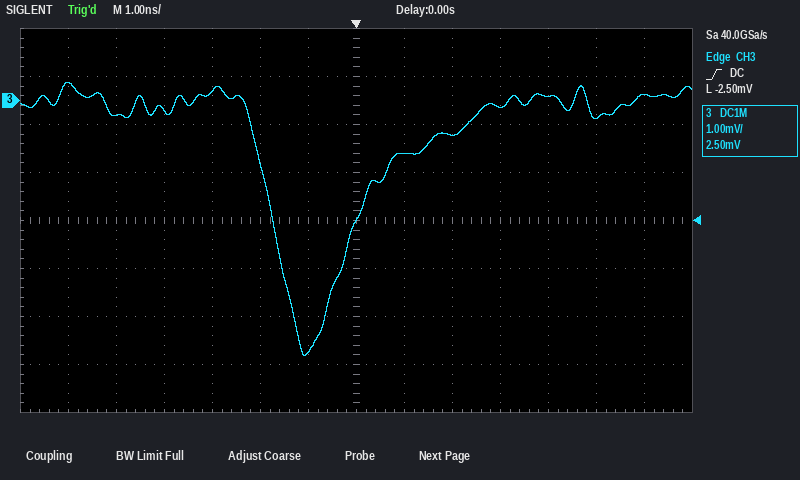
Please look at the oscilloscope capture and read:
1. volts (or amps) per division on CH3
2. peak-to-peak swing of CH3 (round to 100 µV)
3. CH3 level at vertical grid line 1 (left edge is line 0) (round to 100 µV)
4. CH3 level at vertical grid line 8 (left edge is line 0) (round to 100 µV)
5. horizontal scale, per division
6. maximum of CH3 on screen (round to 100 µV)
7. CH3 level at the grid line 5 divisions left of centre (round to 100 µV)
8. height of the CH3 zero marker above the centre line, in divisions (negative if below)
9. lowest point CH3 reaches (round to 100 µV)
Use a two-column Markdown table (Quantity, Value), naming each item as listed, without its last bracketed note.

| Quantity | Value |
|---|---|
| volts (or amps) per division on CH3 | 1 mV |
| peak-to-peak swing of CH3 | 5.7 mV |
| CH3 level at vertical grid line 1 (left edge is line 0) | 400 µV |
| CH3 level at vertical grid line 8 (left edge is line 0) | -1.1 mV |
| horizontal scale, per division | 1 ns |
| maximum of CH3 on screen | 400 µV |
| CH3 level at the grid line 5 divisions left of centre | -300 µV |
| height of the CH3 zero marker above the centre line, in divisions | +2.5 div |
| lowest point CH3 reaches | -5.3 mV |
